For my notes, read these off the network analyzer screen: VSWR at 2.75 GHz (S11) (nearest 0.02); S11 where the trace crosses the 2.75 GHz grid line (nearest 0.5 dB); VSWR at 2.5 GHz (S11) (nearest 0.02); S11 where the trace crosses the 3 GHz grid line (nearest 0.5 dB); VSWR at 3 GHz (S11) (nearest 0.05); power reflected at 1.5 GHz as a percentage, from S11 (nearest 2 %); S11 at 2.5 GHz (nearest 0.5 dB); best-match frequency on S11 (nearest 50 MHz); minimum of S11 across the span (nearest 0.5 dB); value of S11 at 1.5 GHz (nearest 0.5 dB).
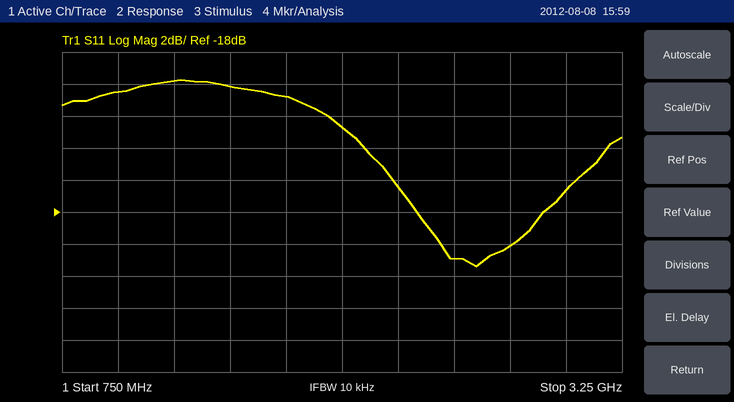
1.22
-20.0 dB
1.20
-16.5 dB
1.35
10 %
-21.0 dB
2.60 GHz
-21.5 dB
-10.0 dB
